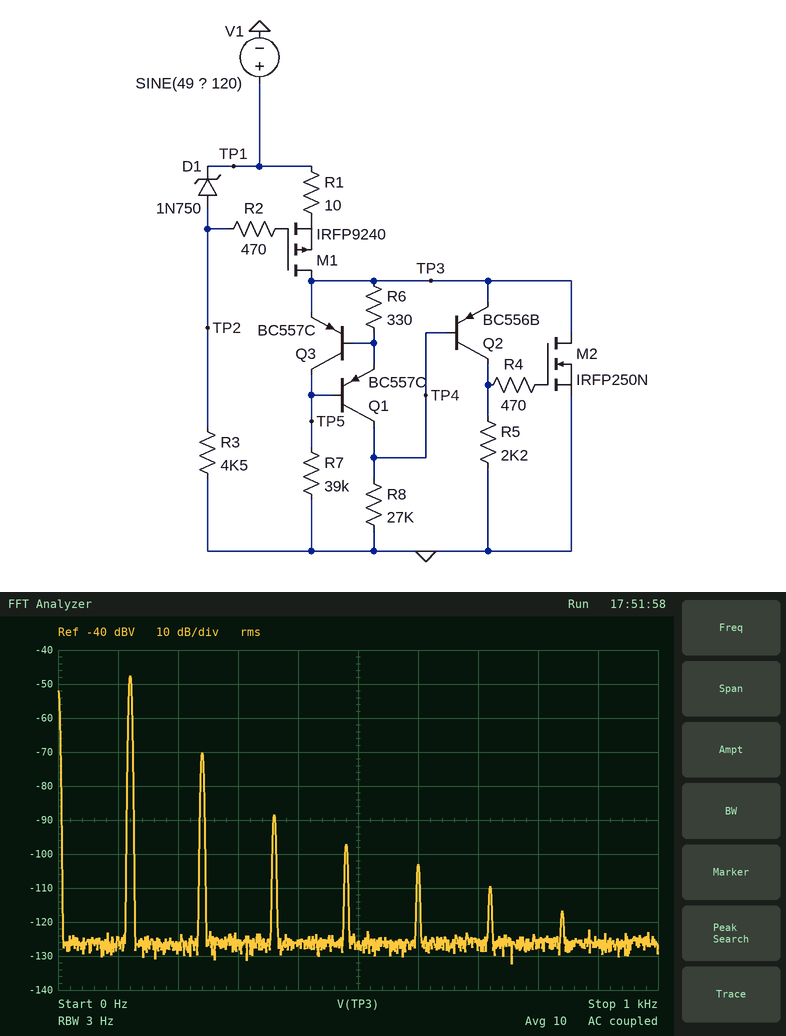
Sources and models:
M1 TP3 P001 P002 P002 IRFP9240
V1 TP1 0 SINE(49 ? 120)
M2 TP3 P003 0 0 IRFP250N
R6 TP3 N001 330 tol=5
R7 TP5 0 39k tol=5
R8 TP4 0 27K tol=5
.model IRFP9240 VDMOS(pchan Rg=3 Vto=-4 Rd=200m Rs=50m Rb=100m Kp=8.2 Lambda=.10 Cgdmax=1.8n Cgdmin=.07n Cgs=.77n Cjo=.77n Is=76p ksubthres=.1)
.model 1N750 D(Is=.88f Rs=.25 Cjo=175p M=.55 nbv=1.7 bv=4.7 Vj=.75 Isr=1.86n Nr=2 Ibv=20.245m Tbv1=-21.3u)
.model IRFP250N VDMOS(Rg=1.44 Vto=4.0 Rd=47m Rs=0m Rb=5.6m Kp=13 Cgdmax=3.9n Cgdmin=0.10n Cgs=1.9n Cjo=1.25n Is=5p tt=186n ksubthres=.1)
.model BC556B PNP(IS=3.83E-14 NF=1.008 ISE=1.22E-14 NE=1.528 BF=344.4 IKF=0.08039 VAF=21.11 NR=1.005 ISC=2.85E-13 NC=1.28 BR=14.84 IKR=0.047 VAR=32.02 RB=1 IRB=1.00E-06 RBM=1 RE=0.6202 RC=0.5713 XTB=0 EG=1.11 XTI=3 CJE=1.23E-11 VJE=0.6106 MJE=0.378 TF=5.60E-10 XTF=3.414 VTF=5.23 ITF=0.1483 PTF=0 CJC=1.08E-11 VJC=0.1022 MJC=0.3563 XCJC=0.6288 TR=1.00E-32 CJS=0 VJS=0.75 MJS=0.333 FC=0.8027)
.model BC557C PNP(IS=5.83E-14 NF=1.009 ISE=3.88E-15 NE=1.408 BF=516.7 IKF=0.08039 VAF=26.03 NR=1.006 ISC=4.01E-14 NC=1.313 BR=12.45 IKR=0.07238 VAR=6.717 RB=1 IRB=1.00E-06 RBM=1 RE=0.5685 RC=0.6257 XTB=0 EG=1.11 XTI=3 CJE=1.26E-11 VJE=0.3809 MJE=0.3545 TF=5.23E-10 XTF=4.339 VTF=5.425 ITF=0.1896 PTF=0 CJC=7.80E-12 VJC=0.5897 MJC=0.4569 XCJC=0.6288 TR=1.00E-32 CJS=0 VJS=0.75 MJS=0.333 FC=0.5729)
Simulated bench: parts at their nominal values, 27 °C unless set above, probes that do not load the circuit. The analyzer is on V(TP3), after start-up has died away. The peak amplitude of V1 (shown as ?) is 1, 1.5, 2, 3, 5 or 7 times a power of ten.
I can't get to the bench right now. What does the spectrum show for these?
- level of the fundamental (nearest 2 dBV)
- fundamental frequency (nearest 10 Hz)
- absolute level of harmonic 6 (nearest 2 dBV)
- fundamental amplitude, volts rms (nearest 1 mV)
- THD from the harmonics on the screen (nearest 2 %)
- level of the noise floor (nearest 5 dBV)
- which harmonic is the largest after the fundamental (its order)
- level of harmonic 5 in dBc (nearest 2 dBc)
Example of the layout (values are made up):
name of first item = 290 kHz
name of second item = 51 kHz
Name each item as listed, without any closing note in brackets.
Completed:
level of the fundamental = -48 dBV
fundamental frequency = 120 Hz
absolute level of harmonic 6 = -110 dBV
fundamental amplitude, volts rms = 4 mV
THD from the harmonics on the screen = 8 %
level of the noise floor = -125 dBV
which harmonic is the largest after the fundamental = 2
level of harmonic 5 in dBc = -56 dBc
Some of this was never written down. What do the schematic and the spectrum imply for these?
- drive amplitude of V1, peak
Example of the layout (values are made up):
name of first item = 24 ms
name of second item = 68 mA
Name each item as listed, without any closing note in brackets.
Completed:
drive amplitude of V1, peak = 5 V
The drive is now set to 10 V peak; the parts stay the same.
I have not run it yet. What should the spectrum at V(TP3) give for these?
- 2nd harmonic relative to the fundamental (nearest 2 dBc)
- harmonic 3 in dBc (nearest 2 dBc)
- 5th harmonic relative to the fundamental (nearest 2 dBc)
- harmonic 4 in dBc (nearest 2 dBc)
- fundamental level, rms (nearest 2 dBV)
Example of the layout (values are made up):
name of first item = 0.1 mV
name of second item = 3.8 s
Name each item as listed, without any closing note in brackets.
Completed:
2nd harmonic relative to the fundamental = -2 dBc
harmonic 3 in dBc = -2 dBc
5th harmonic relative to the fundamental = -6 dBc
harmonic 4 in dBc = -4 dBc
fundamental level, rms = -26 dBV
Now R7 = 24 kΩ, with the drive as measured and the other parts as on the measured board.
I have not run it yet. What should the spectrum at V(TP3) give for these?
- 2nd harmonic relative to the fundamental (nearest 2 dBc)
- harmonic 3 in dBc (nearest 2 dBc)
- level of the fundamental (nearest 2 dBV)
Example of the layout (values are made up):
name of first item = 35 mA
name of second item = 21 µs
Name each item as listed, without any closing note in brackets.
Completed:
2nd harmonic relative to the fundamental = -26 dBc
harmonic 3 in dBc = -48 dBc
level of the fundamental = -50 dBV
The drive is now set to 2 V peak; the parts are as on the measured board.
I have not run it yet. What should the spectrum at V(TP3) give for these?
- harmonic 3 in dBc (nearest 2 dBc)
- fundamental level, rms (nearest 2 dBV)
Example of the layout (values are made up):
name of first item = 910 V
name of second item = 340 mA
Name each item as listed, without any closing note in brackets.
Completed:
harmonic 3 in dBc = -58 dBc
fundamental level, rms = -56 dBV
